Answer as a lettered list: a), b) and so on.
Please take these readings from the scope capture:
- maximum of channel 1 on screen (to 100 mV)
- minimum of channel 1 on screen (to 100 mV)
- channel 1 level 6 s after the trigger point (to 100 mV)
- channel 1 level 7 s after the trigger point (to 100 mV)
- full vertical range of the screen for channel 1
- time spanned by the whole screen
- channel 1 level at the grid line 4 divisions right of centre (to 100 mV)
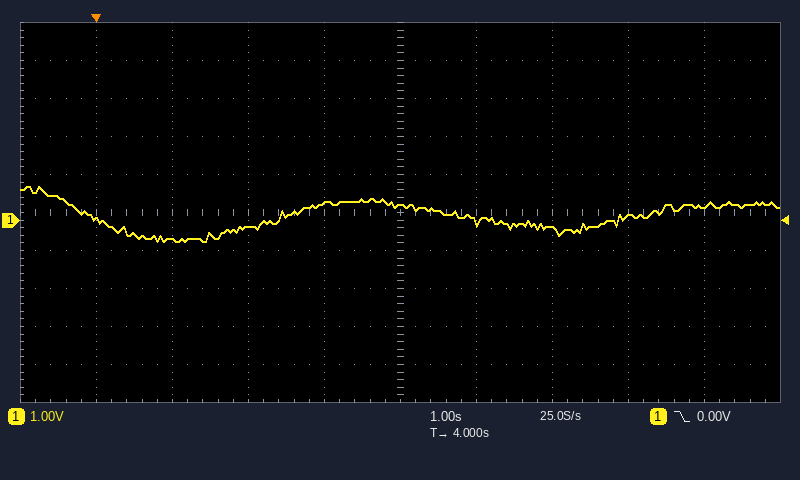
a) 900 mV
b) -600 mV
c) -200 mV
d) 100 mV
e) 10 V
f) 10 s
g) 400 mV
